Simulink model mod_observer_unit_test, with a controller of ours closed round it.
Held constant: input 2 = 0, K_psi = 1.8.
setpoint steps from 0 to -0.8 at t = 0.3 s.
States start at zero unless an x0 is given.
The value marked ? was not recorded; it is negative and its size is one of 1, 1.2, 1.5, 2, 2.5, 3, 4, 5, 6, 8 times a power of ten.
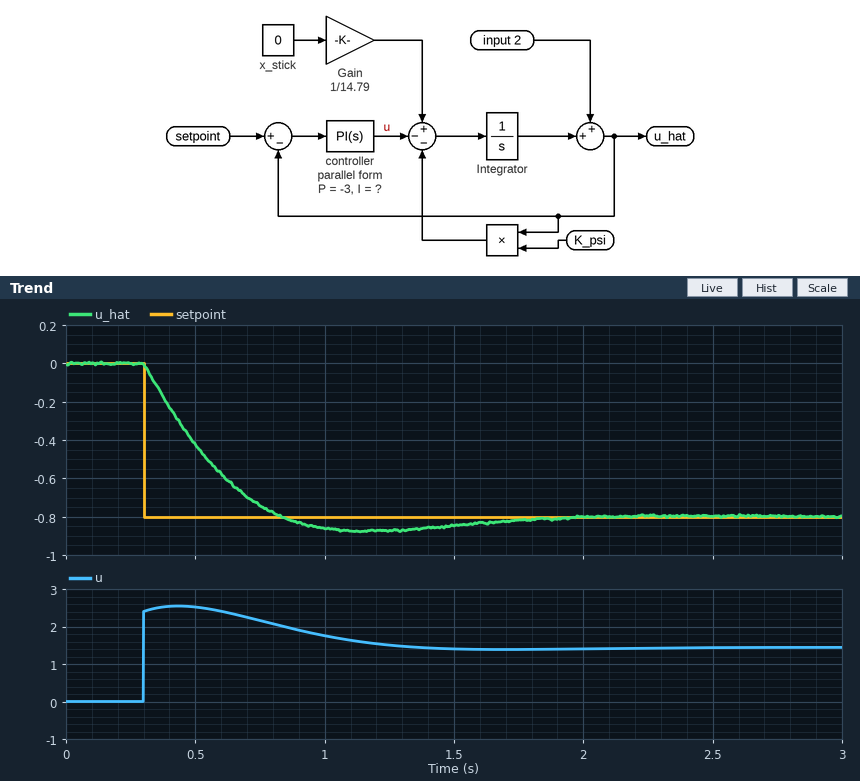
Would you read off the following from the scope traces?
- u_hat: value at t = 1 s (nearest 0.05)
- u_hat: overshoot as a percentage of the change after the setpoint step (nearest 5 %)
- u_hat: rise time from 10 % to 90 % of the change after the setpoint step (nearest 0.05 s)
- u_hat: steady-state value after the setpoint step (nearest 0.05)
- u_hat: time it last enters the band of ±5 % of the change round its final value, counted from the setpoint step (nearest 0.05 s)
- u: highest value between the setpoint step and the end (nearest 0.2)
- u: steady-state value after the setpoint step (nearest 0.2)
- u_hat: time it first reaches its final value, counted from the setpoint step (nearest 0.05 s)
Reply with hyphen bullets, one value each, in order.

- -0.85
- 10 %
- 0.40 s
- -0.80
- 1.25 s
- 2.6
- 1.4
- 0.55 s
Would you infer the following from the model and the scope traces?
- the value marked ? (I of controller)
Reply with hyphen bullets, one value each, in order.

- -12
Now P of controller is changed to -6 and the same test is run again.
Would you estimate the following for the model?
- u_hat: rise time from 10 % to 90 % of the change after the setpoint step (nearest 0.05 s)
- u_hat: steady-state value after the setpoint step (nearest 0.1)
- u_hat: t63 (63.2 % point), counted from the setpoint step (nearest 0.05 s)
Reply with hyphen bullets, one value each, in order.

- 0.35 s
- -0.8
- 0.15 s
